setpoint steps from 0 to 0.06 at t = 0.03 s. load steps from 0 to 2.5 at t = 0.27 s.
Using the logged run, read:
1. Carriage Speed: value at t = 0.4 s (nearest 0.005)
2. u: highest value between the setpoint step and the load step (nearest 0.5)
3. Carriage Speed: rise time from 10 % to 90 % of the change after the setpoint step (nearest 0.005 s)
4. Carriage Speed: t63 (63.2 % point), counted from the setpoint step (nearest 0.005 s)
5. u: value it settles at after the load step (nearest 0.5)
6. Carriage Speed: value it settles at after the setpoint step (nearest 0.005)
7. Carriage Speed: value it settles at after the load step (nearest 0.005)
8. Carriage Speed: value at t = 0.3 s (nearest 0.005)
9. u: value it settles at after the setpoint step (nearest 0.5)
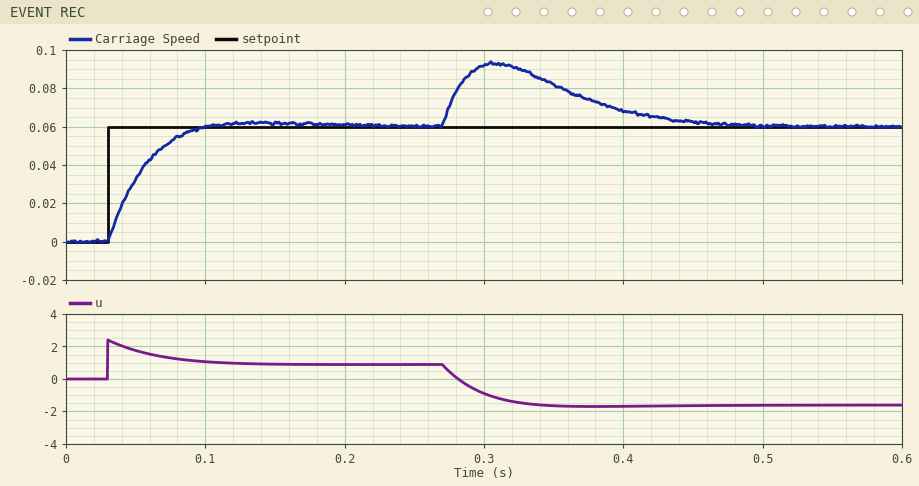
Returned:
0.070
2.5
0.045 s
0.025 s
-1.5
0.060
0.060
0.090
1.0
